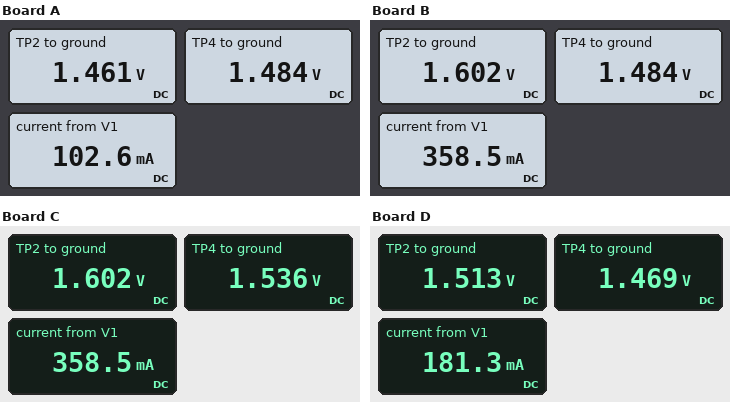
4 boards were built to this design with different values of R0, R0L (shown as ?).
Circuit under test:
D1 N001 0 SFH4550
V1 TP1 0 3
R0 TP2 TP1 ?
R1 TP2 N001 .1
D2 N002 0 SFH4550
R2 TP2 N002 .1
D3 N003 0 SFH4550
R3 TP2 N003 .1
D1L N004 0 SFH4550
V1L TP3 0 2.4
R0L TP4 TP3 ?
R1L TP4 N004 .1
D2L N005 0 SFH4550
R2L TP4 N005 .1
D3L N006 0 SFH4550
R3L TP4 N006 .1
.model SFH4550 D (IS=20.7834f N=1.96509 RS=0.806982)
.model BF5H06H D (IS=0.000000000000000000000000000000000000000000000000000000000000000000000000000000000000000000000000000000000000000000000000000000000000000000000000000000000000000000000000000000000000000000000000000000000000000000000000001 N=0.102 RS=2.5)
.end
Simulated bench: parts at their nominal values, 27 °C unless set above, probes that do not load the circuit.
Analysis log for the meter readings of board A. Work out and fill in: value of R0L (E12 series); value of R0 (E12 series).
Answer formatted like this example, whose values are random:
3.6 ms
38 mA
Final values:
6.8 Ω
15 Ω
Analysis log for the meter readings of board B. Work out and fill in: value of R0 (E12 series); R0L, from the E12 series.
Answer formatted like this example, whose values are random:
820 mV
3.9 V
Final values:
3.9 Ω
6.8 Ω
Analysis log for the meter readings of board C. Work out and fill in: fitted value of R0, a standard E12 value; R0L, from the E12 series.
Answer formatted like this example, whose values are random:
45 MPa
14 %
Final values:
3.9 Ω
3.9 Ω
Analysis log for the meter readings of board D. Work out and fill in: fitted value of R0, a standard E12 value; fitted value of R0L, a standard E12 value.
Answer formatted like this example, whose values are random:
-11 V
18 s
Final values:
8.2 Ω
8.2 Ω
